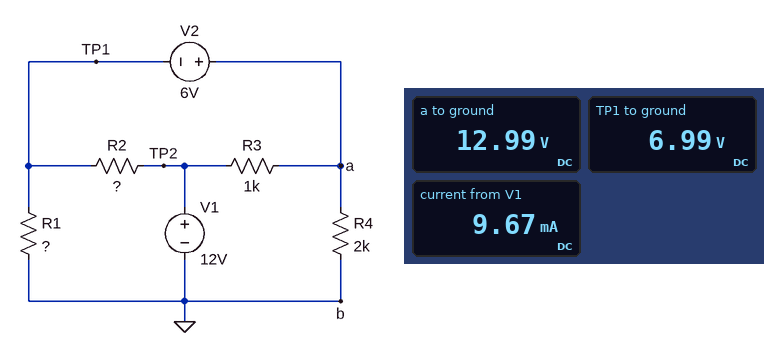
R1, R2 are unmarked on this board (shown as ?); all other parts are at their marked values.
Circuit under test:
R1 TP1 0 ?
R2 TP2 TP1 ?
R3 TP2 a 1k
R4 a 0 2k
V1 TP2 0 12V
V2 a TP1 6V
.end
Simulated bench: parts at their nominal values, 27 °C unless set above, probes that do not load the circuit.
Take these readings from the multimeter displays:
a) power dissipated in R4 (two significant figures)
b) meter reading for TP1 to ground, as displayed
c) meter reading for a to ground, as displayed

84 mW
6.99 V
12.99 V
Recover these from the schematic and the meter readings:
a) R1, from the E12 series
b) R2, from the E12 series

2.2 kΩ
470 Ω
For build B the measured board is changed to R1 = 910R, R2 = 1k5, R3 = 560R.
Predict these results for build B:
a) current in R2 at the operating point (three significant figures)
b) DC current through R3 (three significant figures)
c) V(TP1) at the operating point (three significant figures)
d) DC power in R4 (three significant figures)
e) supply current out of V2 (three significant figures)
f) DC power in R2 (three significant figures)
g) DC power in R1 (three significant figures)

5.41 mA
3.79 mA
3.88 V
48.8 mW
1.15 mA
44.0 mW
16.5 mW
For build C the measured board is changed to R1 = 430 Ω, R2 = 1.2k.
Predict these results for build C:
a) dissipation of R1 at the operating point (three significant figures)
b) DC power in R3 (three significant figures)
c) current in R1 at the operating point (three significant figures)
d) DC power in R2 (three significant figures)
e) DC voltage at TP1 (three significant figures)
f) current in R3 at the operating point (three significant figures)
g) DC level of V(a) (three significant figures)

18.1 mW
10.3 mW
6.49 mA
70.7 mW
2.79 V
3.21 mA
8.79 V
